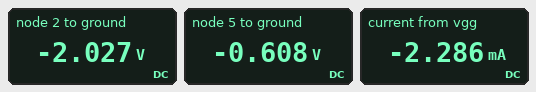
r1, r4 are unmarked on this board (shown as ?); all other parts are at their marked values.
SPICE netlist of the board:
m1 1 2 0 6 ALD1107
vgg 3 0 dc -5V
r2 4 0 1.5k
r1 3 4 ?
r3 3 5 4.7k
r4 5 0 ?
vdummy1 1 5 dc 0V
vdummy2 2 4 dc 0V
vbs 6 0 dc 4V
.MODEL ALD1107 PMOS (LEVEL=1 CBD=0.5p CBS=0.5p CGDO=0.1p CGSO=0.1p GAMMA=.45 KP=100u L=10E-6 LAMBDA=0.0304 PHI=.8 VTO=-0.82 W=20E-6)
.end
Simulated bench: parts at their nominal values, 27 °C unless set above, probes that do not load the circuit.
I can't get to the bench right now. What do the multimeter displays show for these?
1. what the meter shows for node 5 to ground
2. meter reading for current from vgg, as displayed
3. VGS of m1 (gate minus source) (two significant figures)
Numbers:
-0.608 V
-2.286 mA
-2.0 V
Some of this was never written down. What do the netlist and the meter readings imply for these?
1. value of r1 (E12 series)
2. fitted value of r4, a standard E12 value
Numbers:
2.2 kΩ
680 Ω
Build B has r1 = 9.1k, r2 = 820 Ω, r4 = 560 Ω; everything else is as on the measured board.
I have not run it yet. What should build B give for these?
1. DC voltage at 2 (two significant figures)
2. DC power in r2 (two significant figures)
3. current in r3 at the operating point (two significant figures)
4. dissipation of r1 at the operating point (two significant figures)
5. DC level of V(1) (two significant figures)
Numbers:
-410 mV
210 µW
950 µA
2.3 mW
-530 mV
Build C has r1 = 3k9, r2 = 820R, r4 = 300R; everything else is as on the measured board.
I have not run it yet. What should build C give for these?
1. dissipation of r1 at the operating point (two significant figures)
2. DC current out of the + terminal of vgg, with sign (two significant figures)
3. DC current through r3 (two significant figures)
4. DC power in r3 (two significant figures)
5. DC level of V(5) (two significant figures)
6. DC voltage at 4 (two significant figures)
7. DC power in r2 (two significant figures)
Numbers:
4.4 mW
-2.1 mA
1.0 mA
4.7 mW
-300 mV
-870 mV
920 µW
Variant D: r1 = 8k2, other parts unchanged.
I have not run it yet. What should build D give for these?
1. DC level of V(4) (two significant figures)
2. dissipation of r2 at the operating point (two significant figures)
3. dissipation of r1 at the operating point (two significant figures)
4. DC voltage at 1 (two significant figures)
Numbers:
-770 mV
400 µW
2.2 mW
-630 mV
